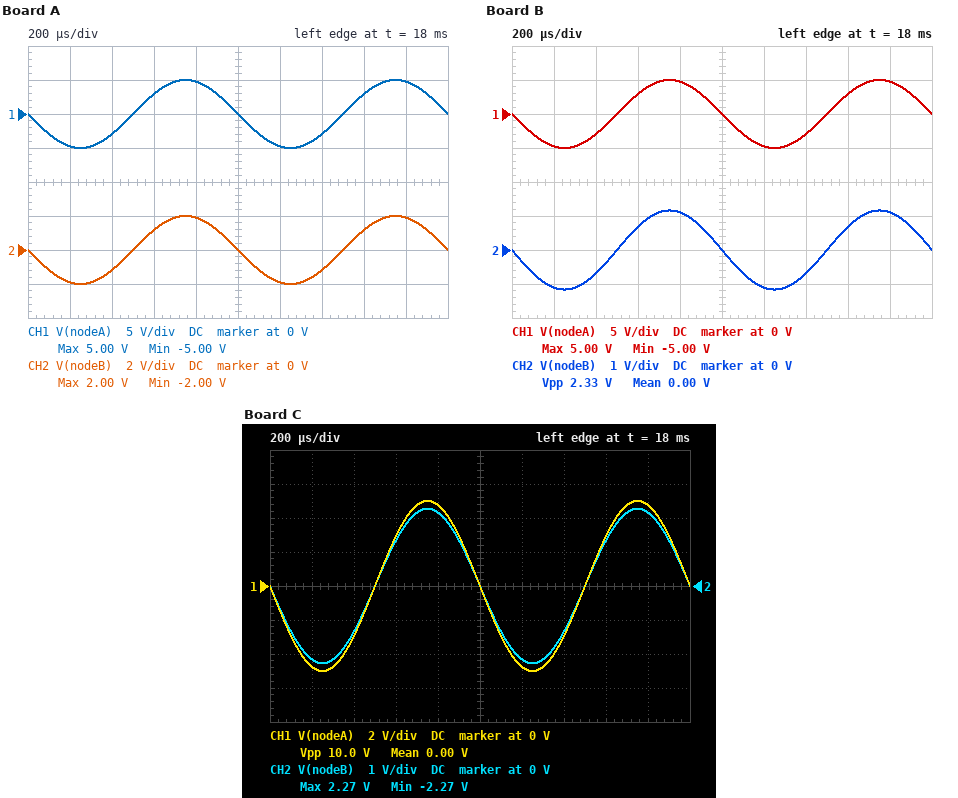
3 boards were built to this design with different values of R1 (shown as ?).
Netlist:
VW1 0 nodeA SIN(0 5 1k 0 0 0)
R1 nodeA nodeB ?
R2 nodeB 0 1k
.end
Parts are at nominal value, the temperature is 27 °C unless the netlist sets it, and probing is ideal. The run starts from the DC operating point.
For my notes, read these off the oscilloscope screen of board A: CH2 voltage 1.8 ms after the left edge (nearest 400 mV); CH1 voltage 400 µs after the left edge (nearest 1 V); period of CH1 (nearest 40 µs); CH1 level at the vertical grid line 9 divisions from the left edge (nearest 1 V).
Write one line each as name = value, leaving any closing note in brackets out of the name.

CH2 voltage 1.8 ms after the left edge = 2.0 V
CH1 voltage 400 µs after the left edge = -3 V
period of CH1 = 1.00 ms
CH1 level at the vertical grid line 9 divisions from the left edge = 5 V
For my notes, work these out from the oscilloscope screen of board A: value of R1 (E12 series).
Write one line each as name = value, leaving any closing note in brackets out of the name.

value of R1 = 1.5 kΩ
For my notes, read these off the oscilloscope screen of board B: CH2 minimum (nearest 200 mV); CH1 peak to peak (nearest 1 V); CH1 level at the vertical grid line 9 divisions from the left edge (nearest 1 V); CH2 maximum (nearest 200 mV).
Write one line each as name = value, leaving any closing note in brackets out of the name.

CH2 minimum = -1.2 V
CH1 peak to peak = 10 V
CH1 level at the vertical grid line 9 divisions from the left edge = 5 V
CH2 maximum = 1.2 V
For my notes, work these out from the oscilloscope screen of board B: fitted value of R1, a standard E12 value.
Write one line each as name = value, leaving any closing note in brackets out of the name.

fitted value of R1, a standard E12 value = 3.3 kΩ
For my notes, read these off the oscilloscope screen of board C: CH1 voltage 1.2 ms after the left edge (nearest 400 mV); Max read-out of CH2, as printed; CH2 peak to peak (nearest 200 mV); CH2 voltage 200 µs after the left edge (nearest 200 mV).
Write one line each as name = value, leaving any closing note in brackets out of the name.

CH1 voltage 1.2 ms after the left edge = -4.8 V
Max read-out of CH2, as printed = 2.27 V
CH2 peak to peak = 4.6 V
CH2 voltage 200 µs after the left edge = -2.2 V
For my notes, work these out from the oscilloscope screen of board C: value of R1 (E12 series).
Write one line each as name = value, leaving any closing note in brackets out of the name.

value of R1 = 1.2 kΩ
